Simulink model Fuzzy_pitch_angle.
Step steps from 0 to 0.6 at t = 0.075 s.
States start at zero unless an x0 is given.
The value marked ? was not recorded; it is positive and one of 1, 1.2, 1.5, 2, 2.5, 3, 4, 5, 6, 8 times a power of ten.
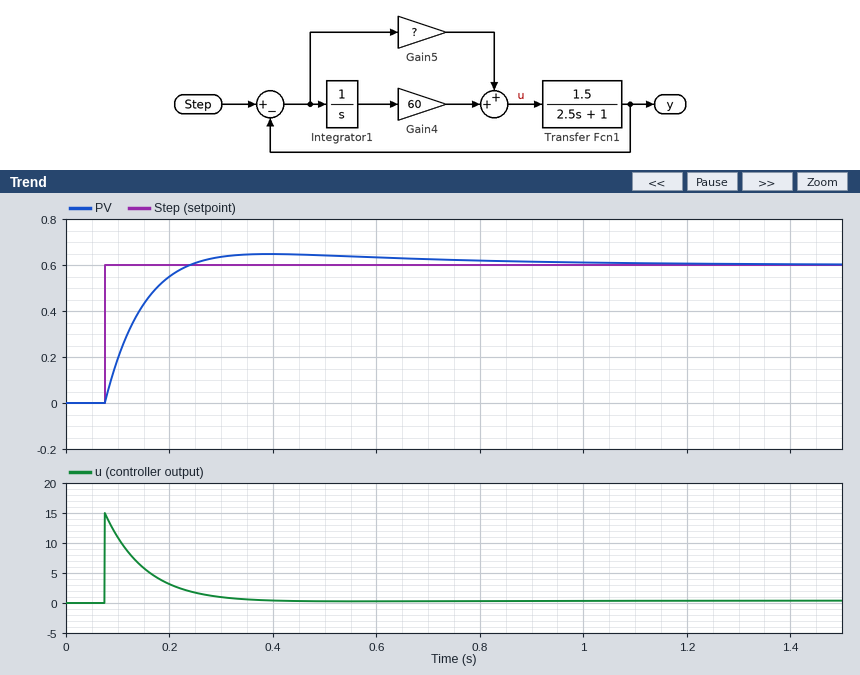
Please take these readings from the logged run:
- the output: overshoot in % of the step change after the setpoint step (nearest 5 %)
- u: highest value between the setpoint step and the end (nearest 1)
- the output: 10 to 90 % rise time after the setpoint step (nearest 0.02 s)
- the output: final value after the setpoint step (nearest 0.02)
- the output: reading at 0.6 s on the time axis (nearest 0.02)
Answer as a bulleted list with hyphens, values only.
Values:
- 10 %
- 15
- 0.12 s
- 0.60
- 0.64
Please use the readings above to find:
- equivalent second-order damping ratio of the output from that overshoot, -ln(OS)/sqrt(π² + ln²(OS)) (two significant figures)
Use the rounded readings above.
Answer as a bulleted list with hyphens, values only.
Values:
- 0.59
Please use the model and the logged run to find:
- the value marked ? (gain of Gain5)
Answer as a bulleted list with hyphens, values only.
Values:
- 25
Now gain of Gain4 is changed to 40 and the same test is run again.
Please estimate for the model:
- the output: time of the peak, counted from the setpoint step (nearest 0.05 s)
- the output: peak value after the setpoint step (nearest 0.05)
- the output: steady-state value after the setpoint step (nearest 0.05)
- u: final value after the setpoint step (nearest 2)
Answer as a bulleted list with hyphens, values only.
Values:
- 0.35 s
- 0.65
- 0.60
- 0
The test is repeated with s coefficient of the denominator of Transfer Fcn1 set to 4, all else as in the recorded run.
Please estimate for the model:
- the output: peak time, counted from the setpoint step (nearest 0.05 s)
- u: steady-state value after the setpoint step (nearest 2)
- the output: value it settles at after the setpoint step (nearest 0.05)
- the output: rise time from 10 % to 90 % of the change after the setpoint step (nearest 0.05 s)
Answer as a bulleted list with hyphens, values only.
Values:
- 0.45 s
- 0
- 0.60
- 0.15 s
